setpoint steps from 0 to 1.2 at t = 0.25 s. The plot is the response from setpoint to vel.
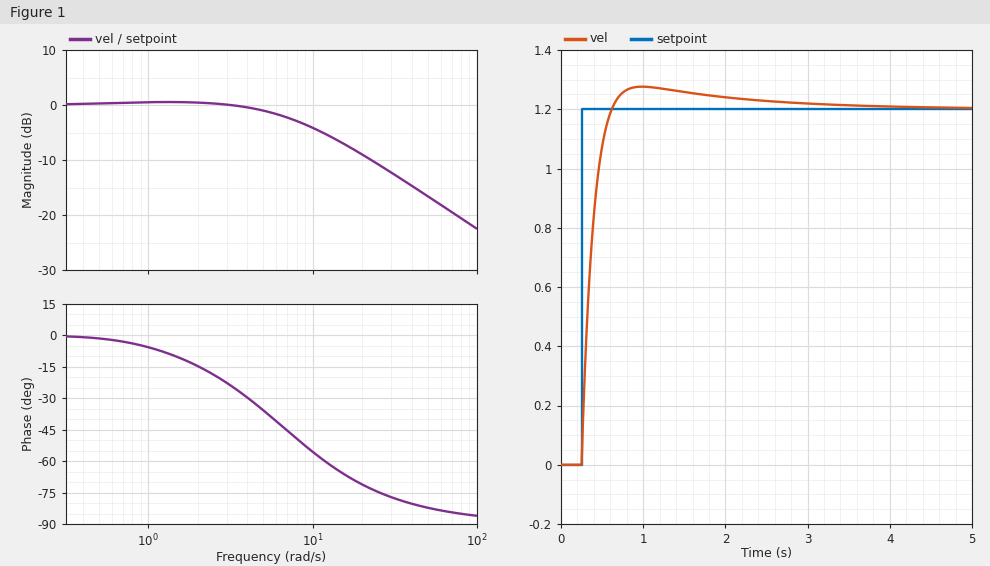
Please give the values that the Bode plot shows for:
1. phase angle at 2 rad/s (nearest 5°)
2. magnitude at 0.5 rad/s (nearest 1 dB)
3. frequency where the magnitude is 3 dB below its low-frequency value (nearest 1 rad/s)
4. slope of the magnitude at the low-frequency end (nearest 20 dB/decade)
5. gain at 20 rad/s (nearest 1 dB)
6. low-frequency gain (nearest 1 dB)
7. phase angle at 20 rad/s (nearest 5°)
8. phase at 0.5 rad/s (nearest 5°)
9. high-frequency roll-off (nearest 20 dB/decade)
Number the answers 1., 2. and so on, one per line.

1. -15°
2. 0 dB
3. 8 rad/s
4. 0 dB/decade
5. -9 dB
6. 0 dB
7. -70°
8. 0°
9. -20 dB/decade
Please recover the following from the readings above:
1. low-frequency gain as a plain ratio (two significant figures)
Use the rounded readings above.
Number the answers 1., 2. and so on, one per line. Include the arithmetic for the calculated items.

1. 10^(0 / 20) = 1.0
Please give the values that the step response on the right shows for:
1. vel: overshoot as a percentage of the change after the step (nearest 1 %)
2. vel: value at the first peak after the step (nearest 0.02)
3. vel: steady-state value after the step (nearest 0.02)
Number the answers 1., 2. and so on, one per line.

1. 6 %
2. 1.28
3. 1.20
